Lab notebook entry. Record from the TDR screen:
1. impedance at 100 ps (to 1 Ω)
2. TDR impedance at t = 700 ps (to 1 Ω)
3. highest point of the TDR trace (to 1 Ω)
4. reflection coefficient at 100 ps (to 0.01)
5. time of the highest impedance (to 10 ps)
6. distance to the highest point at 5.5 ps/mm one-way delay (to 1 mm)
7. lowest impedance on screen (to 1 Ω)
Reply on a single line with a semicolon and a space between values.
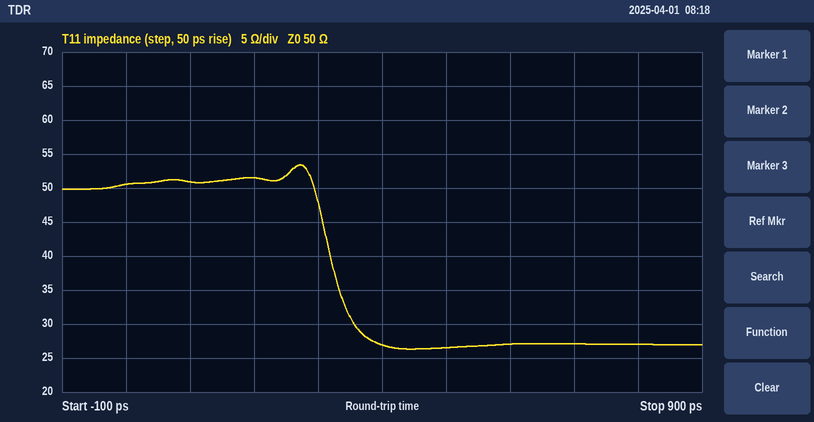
51 Ω; 27 Ω; 53 Ω; +0.01; 270 ps; 25 mm; 26 Ω
